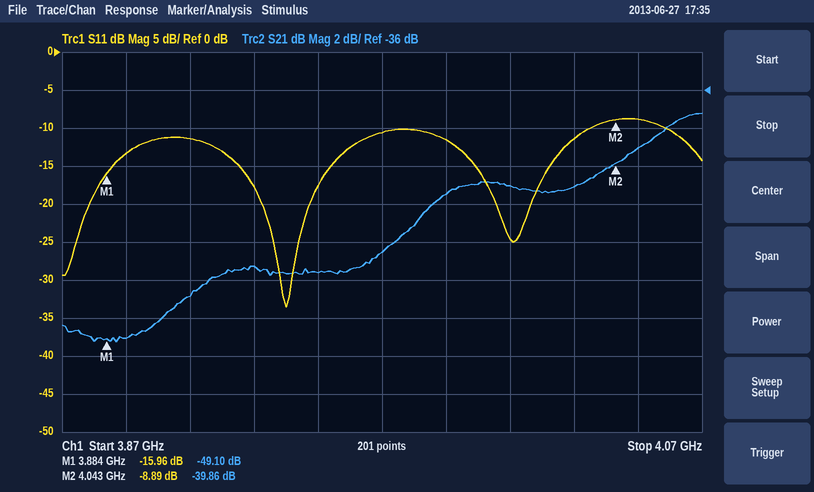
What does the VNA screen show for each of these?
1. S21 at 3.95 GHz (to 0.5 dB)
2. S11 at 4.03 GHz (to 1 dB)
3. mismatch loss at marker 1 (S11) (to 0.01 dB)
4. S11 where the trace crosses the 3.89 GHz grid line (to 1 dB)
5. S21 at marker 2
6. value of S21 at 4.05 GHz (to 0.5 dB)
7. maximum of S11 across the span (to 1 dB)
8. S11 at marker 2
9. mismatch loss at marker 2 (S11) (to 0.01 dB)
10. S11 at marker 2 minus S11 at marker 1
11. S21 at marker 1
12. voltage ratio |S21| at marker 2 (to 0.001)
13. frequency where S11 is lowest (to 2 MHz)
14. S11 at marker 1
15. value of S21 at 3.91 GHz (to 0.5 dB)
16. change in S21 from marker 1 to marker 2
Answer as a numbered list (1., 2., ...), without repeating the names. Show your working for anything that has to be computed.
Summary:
1. -45.5 dB
2. -11 dB
3. −10 log10(1 − 10^(-15.96/10)) ≈ 0.11 dB
4. -13 dB
5. -39.86 dB
6. -39.0 dB
7. -9 dB
8. -8.89 dB
9. −10 log10(1 − 10^(-8.89/10)) ≈ 0.60 dB
10. -8.89 − (-15.96) = 7.07 dB
11. -49.10 dB
12. 10^(-39.86/20) ≈ 0.010
13. 3.940 GHz
14. -15.96 dB
15. -47.0 dB
16. -39.86 − (-49.1) = 9.24 dB
